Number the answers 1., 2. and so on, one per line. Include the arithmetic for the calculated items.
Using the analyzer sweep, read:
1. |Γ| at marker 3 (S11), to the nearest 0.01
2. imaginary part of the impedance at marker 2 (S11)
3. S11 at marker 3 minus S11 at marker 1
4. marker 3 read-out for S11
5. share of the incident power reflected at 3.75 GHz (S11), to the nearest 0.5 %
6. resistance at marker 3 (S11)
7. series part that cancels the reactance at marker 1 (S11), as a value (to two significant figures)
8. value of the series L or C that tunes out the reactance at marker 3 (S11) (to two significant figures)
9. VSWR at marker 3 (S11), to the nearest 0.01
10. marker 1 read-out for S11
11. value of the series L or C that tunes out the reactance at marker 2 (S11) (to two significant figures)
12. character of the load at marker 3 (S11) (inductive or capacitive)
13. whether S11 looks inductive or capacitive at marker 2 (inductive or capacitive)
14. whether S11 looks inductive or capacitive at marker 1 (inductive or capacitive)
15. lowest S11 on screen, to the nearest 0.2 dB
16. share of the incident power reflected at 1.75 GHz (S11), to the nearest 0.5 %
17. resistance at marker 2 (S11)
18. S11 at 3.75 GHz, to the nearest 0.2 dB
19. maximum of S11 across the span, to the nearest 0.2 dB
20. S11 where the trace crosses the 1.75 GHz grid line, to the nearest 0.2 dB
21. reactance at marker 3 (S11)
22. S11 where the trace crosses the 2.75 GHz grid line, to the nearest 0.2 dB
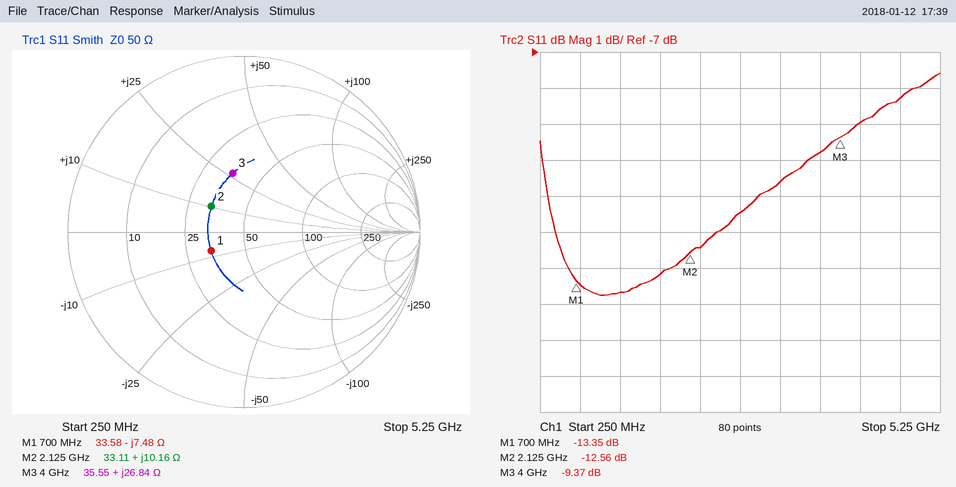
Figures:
1. 0.34
2. +10.16 Ω
3. -9.37 − (-13.35) = 3.98 dB
4. -9.37 dB
5. 10^(-9.8/10) ≈ 10.5 %
6. 35.55 Ω
7. L = 7.48 Ω/(2π × 700 MHz) ≈ 1.7 nH
8. C = 1/(2π × 4 GHz × 26.84 Ω) ≈ 1.5 pF
9. (1 + 0.3400)/(1 − 0.3400) ≈ 2.03
10. -13.35 dB
11. C = 1/(2π × 2.125 GHz × 10.16 Ω) ≈ 7.4 pF
12. inductive
13. inductive
14. capacitive
15. -13.8 dB
16. 10^(-13.2/10) ≈ 4.79 %, so 5.0 % to the nearest 0.5 %
17. 33.11 Ω
18. -9.8 dB
19. -7.6 dB
20. -13.2 dB
21. +26.84 Ω
22. -11.4 dB
